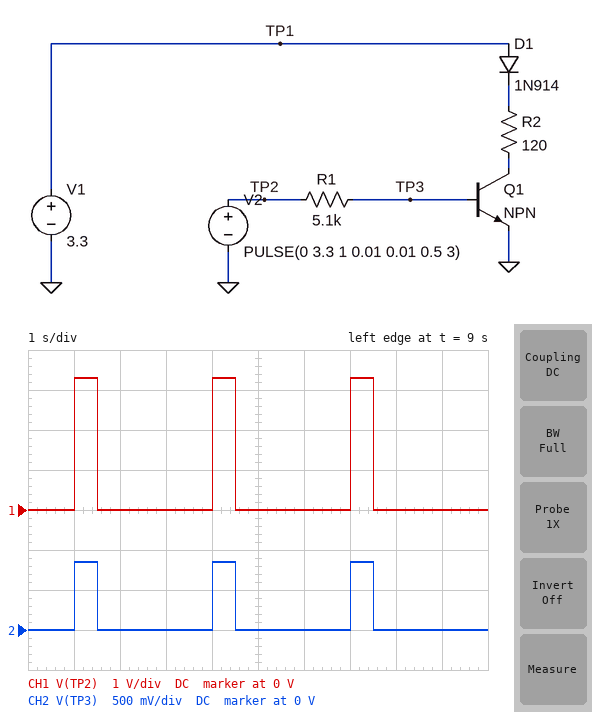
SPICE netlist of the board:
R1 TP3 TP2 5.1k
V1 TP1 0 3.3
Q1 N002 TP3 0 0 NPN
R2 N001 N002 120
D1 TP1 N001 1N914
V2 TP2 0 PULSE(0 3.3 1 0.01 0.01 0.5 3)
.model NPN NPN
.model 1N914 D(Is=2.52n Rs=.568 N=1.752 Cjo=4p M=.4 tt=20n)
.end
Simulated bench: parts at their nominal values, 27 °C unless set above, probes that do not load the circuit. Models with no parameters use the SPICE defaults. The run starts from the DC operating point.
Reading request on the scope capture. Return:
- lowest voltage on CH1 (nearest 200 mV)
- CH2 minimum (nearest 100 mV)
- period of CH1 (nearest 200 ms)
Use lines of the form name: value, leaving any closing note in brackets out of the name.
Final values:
lowest voltage on CH1: 0 V
CH2 minimum: 0 V
period of CH1: 3.0 s
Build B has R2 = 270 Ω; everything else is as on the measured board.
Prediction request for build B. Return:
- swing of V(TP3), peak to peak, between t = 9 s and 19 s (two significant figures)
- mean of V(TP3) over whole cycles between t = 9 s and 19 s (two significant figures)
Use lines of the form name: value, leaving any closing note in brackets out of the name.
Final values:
swing of V(TP3), peak to peak, between t = 9 s and 19 s: 830 mV
mean of V(TP3) over whole cycles between t = 9 s and 19 s: 140 mV
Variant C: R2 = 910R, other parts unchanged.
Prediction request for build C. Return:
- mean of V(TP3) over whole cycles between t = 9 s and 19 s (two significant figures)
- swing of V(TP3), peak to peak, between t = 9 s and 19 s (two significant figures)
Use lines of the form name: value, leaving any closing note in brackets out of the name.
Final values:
mean of V(TP3) over whole cycles between t = 9 s and 19 s: 140 mV
swing of V(TP3), peak to peak, between t = 9 s and 19 s: 810 mV
